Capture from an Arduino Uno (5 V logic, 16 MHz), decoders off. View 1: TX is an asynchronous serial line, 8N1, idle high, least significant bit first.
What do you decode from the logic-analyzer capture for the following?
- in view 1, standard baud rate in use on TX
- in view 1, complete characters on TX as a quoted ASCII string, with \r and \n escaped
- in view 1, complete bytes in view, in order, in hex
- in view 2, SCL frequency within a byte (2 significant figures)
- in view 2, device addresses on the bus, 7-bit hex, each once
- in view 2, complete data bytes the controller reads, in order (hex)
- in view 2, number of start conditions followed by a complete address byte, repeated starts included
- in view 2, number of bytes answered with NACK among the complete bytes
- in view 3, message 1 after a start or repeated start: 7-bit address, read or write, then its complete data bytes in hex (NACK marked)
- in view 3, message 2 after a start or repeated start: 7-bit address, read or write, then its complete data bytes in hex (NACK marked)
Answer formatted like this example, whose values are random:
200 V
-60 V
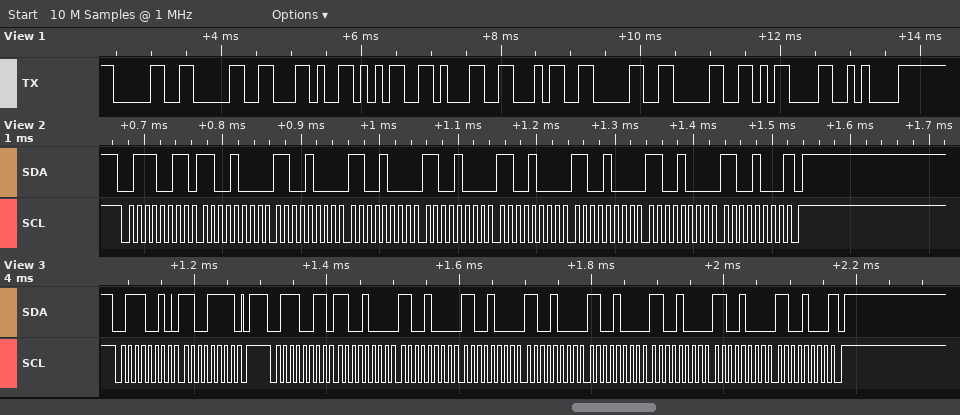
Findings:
9600 baud
"00,51400\r\n"
30 30 2C 35 31 34 30 30 0D 0A
100 kHz
0x39
C8 C8 C8 C8 C8 C8 C8 C8
1
1
0x39 write: CF
0x39 read: C8 C8 C8 C8 C8 C8 C8 C8 NACK
